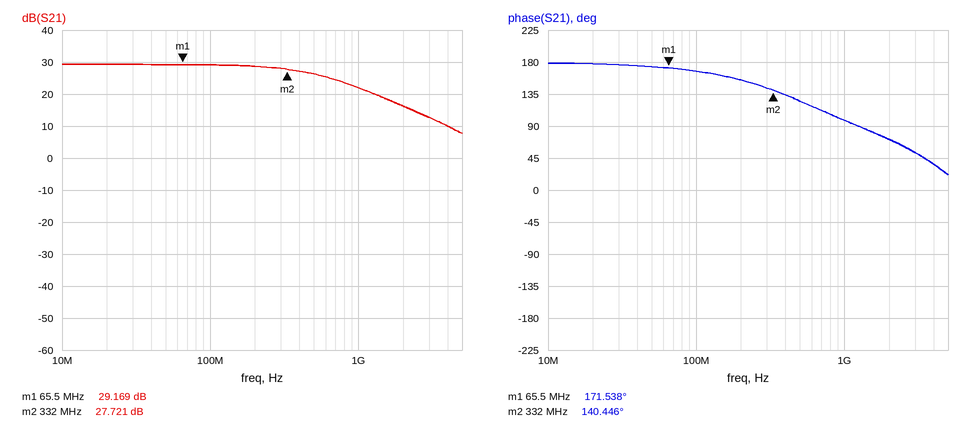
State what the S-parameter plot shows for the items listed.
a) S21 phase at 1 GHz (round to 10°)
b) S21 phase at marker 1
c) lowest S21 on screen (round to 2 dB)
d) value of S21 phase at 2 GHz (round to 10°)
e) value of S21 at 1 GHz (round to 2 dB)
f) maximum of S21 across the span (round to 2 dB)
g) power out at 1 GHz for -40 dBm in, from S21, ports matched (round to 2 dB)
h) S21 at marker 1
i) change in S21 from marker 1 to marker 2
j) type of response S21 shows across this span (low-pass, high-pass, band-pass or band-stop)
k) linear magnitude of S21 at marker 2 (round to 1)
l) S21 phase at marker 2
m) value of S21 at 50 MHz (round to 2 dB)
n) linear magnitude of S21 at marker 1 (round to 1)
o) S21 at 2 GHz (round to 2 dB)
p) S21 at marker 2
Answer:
100°
171.538°
8 dB
70°
22 dB
30 dB
-18 dBm
29.169 dB
-1.448 dB
low-pass
24
140.446°
30 dB
29
16 dB
27.721 dB
